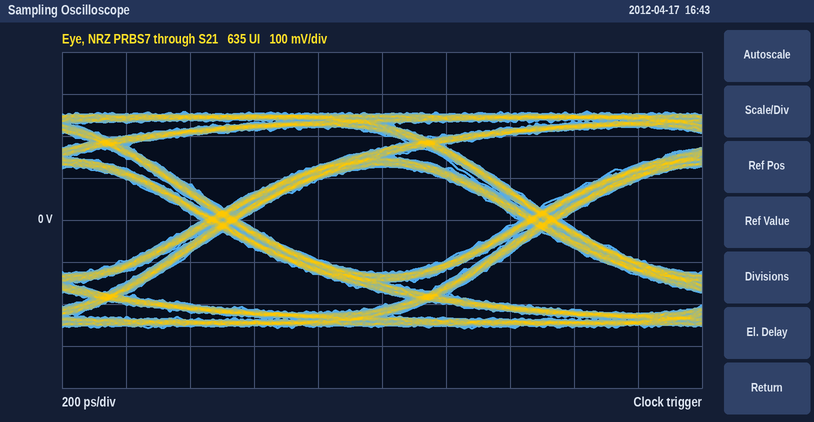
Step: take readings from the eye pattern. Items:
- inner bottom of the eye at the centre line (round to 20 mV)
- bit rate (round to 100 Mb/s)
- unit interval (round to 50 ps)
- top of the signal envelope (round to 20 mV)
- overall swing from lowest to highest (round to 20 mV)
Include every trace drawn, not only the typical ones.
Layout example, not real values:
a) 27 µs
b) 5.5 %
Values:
a) -120 mV
b) 1.0 Gb/s
c) 1.00 ns
d) 260 mV
e) 520 mV
